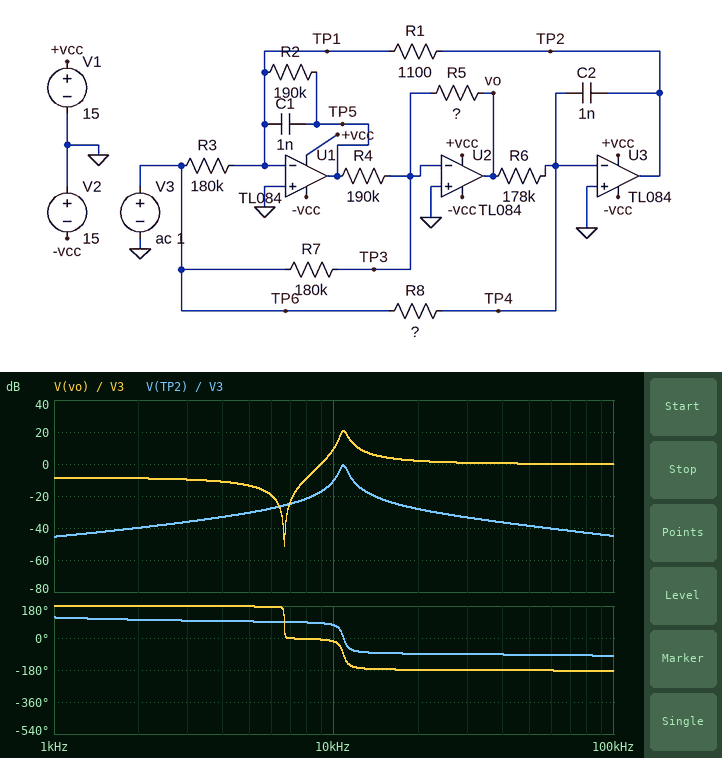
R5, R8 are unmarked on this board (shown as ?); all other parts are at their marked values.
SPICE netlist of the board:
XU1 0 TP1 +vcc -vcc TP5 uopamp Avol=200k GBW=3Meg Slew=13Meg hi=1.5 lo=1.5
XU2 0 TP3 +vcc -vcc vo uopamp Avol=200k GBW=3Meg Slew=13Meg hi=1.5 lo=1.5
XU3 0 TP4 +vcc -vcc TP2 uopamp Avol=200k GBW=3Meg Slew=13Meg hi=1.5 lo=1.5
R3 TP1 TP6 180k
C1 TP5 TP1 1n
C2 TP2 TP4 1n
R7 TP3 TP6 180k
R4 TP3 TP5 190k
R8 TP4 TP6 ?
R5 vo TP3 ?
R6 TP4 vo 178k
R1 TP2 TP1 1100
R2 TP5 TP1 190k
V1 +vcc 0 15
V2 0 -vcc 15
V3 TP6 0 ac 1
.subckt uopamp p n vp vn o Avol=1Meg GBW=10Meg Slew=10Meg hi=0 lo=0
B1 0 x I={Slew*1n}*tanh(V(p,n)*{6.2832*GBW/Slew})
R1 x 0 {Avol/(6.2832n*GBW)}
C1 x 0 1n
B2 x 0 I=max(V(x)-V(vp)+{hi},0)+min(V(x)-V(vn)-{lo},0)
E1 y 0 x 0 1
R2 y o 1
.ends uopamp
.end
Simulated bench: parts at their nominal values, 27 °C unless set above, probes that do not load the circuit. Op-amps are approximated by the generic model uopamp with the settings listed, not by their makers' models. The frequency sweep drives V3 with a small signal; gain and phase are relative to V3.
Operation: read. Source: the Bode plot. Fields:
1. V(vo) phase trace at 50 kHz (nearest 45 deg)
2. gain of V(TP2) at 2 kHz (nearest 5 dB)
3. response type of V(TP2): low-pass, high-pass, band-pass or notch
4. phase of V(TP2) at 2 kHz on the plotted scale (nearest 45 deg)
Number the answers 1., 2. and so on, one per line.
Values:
1. -180 deg
2. -40 dB
3. band-pass
4. 90 deg
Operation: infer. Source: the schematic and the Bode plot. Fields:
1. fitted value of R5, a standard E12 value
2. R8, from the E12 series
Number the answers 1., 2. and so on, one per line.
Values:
1. 180 kΩ
2. 470 kΩ
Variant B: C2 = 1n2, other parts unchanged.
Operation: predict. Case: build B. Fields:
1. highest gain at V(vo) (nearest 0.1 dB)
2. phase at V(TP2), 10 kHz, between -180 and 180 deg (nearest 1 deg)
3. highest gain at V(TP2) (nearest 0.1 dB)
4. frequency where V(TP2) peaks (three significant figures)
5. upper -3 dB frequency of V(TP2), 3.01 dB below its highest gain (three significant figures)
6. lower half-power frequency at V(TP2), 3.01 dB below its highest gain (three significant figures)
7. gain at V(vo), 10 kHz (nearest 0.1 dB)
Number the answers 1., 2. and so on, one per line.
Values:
1. 19.6 dB
2. -21 deg
3. -2.8 dB
4. 9.87 kHz
5. 10.2 kHz
6. 9.55 kHz
7. 19.2 dB
